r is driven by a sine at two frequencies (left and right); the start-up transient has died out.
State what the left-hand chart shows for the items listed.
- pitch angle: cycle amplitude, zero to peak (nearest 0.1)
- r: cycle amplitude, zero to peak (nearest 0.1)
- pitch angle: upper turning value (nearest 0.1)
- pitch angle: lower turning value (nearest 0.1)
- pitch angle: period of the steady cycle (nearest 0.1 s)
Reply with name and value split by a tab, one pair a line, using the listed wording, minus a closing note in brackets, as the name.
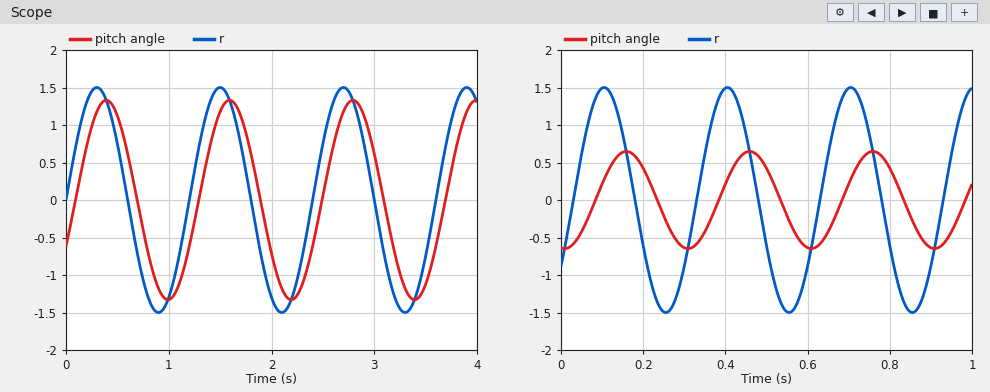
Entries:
pitch angle: cycle amplitude, zero to peak	1.3
r: cycle amplitude, zero to peak	1.5
pitch angle: upper turning value	1.3
pitch angle: lower turning value	-1.3
pitch angle: period of the steady cycle	1.2 s
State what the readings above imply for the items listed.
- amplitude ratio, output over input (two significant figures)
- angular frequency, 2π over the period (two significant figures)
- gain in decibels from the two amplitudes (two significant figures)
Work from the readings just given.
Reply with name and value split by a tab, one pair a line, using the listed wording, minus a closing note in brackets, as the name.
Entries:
amplitude ratio, output over input	0.87
angular frequency, 2π over the period	5.2 rad/s
gain in decibels from the two amplitudes	-1.2 dB
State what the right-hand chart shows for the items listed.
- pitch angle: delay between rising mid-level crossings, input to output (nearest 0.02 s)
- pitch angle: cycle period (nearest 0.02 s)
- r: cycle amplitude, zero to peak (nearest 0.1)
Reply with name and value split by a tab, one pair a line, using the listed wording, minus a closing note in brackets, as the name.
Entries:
pitch angle: delay between rising mid-level crossings, input to output	0.06 s
pitch angle: cycle period	0.30 s
r: cycle amplitude, zero to peak	1.5
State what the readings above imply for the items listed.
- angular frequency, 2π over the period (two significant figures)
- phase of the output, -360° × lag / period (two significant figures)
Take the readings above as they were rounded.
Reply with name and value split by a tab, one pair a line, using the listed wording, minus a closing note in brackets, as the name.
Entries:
angular frequency, 2π over the period	21 rad/s
phase of the output, -360° × lag / period	-72°
